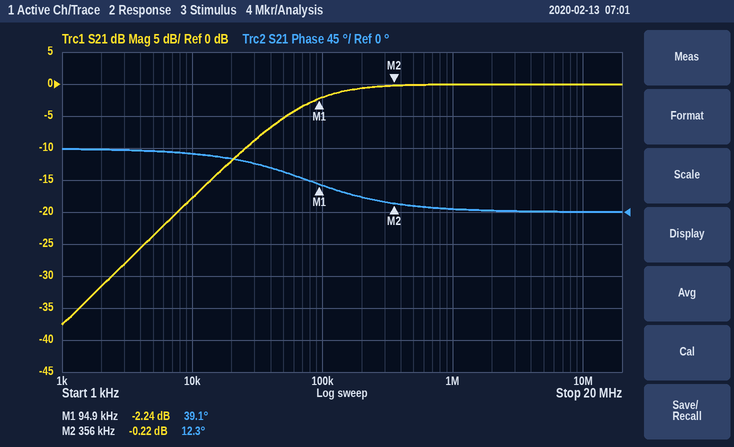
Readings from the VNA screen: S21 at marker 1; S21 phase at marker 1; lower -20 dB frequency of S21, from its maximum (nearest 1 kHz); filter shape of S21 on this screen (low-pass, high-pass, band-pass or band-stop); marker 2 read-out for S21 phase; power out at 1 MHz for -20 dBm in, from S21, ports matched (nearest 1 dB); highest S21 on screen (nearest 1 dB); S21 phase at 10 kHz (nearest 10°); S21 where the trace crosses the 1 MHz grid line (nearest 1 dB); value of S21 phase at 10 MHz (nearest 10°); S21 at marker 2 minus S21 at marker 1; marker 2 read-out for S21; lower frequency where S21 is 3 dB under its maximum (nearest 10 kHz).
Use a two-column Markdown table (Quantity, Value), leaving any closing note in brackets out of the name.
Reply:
| Quantity | Value |
|---|---|
| S21 at marker 1 | -2.24 dB |
| S21 phase at marker 1 | 39.1° |
| lower -20 dB frequency of S21, from its maximum | 8 kHz |
| filter shape of S21 on this screen | high-pass |
| marker 2 read-out for S21 phase | 12.3° |
| power out at 1 MHz for -20 dBm in, from S21, ports matched | -20 dBm |
| highest S21 on screen | 0 dB |
| S21 phase at 10 kHz | 80° |
| S21 where the trace crosses the 1 MHz grid line | 0 dB |
| value of S21 phase at 10 MHz | 0° |
| S21 at marker 2 minus S21 at marker 1 | 2.02 dB |
| marker 2 read-out for S21 | -0.22 dB |
| lower frequency where S21 is 3 dB under its maximum | 80 kHz |
